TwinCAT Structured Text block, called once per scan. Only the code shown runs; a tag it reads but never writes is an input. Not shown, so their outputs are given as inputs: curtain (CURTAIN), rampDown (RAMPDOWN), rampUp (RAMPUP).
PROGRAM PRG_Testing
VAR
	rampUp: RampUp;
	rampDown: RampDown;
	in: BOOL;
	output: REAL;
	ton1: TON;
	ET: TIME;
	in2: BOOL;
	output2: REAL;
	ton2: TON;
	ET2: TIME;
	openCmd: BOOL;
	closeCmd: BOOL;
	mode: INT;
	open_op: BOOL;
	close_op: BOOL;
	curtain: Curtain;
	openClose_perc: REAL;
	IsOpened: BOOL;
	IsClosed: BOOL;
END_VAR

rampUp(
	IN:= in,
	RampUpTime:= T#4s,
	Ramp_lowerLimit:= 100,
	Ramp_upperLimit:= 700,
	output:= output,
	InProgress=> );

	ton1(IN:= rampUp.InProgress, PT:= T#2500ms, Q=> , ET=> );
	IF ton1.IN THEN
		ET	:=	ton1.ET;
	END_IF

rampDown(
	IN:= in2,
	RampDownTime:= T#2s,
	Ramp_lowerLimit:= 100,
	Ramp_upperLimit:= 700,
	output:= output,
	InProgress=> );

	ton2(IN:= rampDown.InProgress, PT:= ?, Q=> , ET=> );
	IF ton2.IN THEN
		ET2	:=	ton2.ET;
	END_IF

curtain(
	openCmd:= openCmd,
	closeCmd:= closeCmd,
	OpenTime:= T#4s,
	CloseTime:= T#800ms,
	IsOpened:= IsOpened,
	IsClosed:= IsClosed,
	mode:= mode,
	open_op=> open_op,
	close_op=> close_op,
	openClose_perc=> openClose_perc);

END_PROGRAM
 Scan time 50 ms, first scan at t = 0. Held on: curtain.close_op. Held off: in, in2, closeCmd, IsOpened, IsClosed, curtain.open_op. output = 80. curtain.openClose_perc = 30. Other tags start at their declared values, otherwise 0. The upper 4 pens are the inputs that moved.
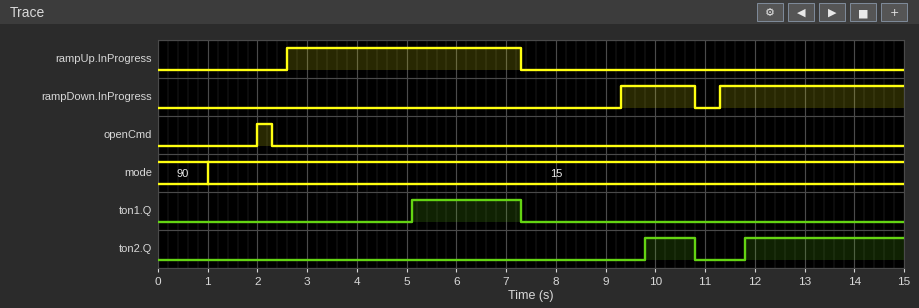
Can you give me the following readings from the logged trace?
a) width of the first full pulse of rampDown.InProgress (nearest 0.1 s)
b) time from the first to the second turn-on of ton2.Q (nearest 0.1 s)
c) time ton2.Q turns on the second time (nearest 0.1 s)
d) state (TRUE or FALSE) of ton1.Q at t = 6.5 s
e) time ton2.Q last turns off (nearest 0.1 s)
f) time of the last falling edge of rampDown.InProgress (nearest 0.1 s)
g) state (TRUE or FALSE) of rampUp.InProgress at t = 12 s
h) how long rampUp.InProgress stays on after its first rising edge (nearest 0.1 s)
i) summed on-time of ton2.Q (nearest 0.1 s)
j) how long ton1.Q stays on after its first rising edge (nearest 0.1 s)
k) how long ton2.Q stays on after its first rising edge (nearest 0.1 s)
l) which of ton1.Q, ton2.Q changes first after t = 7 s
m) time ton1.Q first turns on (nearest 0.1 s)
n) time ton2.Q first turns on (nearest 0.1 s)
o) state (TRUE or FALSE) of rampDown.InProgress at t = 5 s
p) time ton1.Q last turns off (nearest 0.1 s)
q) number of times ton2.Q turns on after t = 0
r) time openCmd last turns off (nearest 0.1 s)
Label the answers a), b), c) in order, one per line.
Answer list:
a) 1.5 s
b) 2.0 s
c) 11.8 s
d) TRUE
e) 10.8 s
f) 10.8 s
g) FALSE
h) 4.7 s
i) 4.2 s
j) 2.2 s
k) 1.0 s
l) ton1.Q
m) 5.1 s
n) 9.8 s
o) FALSE
p) 7.3 s
q) 2
r) 2.3 s
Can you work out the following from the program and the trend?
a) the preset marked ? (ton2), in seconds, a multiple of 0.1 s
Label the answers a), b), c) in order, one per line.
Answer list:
a) 0.5 s
